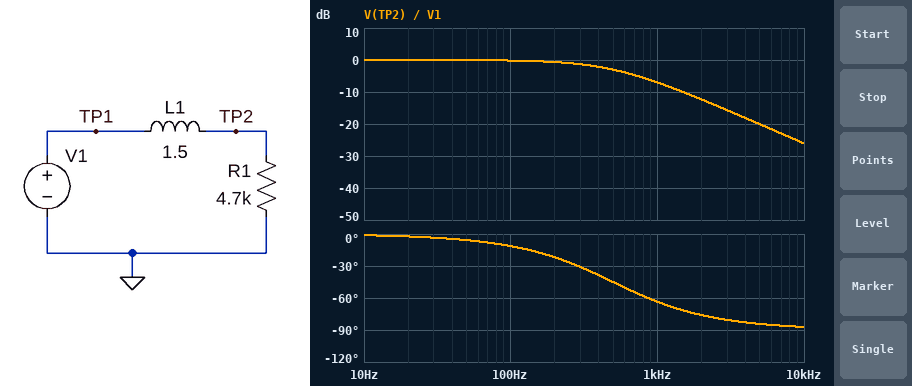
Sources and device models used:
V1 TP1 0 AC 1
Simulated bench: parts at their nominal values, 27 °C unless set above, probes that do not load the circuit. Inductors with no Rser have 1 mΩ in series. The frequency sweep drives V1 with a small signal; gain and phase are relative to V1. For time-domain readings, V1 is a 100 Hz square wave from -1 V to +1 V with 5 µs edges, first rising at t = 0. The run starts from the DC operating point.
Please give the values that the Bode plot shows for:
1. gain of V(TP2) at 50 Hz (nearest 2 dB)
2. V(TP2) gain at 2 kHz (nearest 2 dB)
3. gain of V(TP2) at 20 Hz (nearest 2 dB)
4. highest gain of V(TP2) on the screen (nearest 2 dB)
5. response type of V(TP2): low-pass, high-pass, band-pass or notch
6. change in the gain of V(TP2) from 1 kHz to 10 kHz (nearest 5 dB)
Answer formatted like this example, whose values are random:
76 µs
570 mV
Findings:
0 dB
-12 dB
0 dB
0 dB
low-pass
-20 dB
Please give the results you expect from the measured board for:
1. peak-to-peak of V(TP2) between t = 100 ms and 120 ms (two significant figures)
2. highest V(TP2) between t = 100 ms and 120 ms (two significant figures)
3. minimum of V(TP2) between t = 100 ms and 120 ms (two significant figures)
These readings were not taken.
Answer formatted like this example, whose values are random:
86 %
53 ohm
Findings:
2.0 V
1.0 V
-1.0 V
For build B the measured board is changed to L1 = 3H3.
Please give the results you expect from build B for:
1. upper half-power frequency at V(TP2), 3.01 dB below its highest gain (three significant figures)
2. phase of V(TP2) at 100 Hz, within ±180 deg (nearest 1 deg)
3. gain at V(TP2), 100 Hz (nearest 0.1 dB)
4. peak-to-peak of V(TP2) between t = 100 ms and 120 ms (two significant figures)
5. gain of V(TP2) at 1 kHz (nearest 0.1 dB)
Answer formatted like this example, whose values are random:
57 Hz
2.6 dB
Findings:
227 Hz
-24 deg
-0.8 dB
2.0 V
-13.1 dB
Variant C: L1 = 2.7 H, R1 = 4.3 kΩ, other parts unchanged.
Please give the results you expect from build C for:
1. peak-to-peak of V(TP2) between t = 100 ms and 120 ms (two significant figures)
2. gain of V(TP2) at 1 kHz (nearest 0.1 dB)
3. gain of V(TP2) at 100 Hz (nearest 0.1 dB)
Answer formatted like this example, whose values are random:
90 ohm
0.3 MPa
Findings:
2.0 V
-12.2 dB
-0.6 dB
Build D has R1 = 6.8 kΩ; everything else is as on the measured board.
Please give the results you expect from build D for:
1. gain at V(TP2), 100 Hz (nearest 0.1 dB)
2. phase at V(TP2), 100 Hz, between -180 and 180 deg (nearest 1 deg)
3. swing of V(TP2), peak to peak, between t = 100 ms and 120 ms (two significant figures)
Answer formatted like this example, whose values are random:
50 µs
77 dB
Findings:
-0.1 dB
-8 deg
2.0 V
